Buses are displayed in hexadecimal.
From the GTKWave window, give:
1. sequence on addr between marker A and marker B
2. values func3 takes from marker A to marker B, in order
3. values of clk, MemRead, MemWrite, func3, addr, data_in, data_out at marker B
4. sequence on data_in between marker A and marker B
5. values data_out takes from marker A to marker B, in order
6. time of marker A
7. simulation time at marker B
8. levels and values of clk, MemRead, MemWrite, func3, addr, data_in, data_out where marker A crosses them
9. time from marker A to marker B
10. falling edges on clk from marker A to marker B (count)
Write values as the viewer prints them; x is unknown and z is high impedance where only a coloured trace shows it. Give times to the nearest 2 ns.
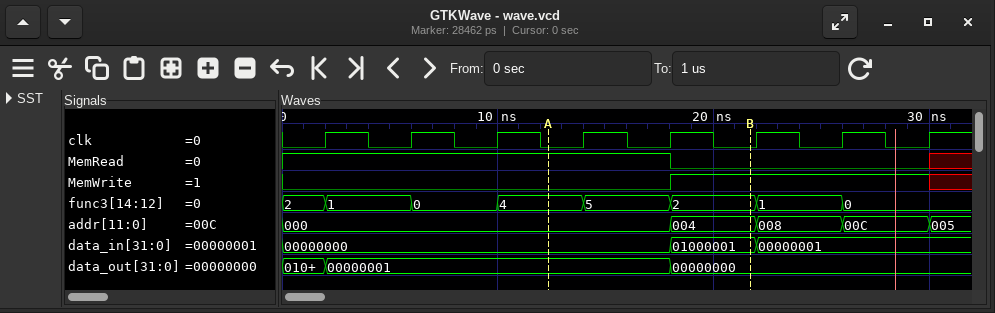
000, 004
4, 5, 2
clk=0, MemRead=0, MemWrite=1, func3=2, addr=004, data_in=01000001, data_out=00000000
00000000, 01000001
00000001, 00000000
12 ns
22 ns
clk=0, MemRead=1, MemWrite=0, func3=4, addr=000, data_in=00000000, data_out=00000001
10 ns
2
